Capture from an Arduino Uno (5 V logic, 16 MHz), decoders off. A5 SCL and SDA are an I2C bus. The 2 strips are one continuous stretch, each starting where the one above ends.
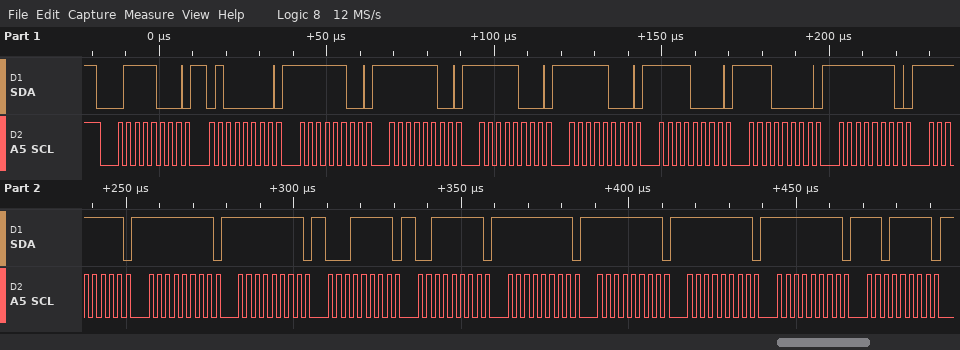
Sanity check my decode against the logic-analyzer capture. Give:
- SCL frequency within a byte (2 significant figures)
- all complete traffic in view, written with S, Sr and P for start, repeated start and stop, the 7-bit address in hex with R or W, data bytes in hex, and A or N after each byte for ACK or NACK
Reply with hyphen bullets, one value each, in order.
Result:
- 400 kHz
- S 3CW A 40 A FC A FC A F8 A F8 A F0 A E0 A FE A FF A FF A FF A 1F A 3F A FF A FF A FF A FF A DF A
